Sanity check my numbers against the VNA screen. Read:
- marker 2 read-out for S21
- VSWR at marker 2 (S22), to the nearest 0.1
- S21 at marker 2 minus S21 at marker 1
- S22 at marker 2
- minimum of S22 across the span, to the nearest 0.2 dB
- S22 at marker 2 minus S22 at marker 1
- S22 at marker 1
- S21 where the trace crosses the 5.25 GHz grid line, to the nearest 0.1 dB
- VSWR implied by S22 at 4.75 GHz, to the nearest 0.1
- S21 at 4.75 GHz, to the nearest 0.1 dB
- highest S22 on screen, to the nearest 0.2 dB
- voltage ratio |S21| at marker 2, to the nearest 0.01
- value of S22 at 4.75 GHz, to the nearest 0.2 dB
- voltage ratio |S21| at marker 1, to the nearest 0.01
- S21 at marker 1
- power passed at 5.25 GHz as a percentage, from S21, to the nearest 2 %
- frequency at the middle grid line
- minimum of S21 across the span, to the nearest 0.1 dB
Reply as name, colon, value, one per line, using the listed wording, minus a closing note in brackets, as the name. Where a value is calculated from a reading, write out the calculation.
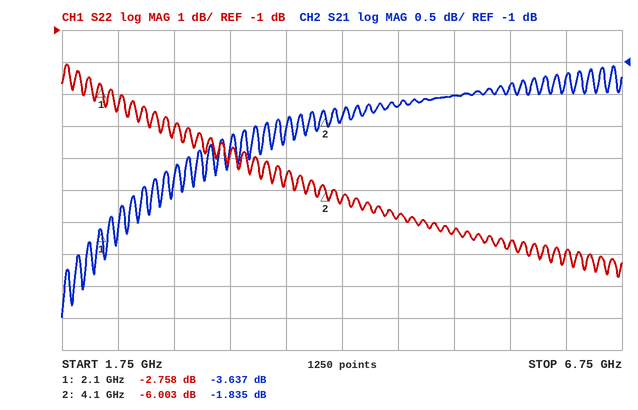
marker 2 read-out for S21: -1.835 dB
VSWR at marker 2 (S22), to the nearest 0.1: (1 + 0.5010)/(1 − 0.5010) ≈ 3.0
S21 at marker 2 minus S21 at marker 1: -1.835 − (-3.637) = 1.802 dB
S22 at marker 2: -6.003 dB
minimum of S22 across the span, to the nearest 0.2 dB: -8.8 dB
S22 at marker 2 minus S22 at marker 1: -6.003 − (-2.758) = -3.245 dB
S22 at marker 1: -2.758 dB
S21 where the trace crosses the 5.25 GHz grid line, to the nearest 0.1 dB: -1.5 dB
VSWR implied by S22 at 4.75 GHz, to the nearest 0.1: |Γ| = 10^(-6.8/20) = 0.4571; VSWR = (1 + 0.4571)/(1 − 0.4571) ≈ 2.7
S21 at 4.75 GHz, to the nearest 0.1 dB: -1.7 dB
highest S22 on screen, to the nearest 0.2 dB: -2.0 dB
voltage ratio |S21| at marker 2, to the nearest 0.01: 10^(-1.835/20) ≈ 0.81
value of S22 at 4.75 GHz, to the nearest 0.2 dB: -6.8 dB
voltage ratio |S21| at marker 1, to the nearest 0.01: 10^(-3.637/20) ≈ 0.66
S21 at marker 1: -3.637 dB
power passed at 5.25 GHz as a percentage, from S21, to the nearest 2 %: 10^(-1.5/10) ≈ 70.8 %, so 70 % to the nearest 2 %
frequency at the middle grid line: 4.25 GHz
minimum of S21 across the span, to the nearest 0.1 dB: -5.0 dB
